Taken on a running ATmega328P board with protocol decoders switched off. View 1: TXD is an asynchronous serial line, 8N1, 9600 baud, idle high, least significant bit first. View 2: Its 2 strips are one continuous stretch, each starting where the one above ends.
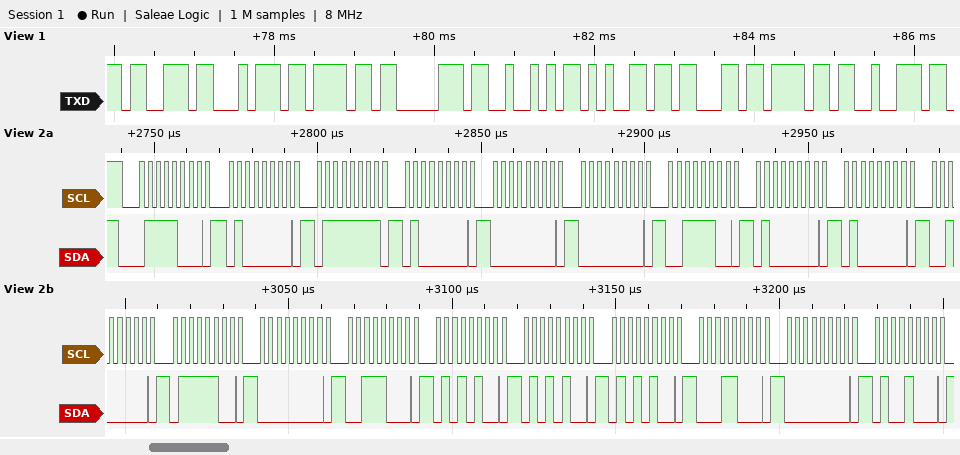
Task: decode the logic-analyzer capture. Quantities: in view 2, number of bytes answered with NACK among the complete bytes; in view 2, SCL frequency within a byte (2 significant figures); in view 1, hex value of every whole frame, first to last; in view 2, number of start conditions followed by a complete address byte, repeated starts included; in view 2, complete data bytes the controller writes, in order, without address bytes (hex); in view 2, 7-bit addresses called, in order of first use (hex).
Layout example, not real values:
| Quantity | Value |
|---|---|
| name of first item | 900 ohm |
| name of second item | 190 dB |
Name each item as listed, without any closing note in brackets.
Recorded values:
| Quantity | Value |
|---|---|
| in view 2, number of bytes answered with NACK among the complete bytes | 0 |
| in view 2, SCL frequency within a byte | 400 kHz |
| in view 1, hex value of every whole frame, first to last | 73 74 6F 70 52 65 63 6F 72 |
| in view 2, number of start conditions followed by a complete address byte, repeated starts included | 1 |
| in view 2, complete data bytes the controller writes, in order, without address bytes | 40 7F 40 00 00 3C 40 40 20 7C 00 38 54 54 54 18 00 48 |
| in view 2, 7-bit addresses called, in order of first use | 0x3C |
